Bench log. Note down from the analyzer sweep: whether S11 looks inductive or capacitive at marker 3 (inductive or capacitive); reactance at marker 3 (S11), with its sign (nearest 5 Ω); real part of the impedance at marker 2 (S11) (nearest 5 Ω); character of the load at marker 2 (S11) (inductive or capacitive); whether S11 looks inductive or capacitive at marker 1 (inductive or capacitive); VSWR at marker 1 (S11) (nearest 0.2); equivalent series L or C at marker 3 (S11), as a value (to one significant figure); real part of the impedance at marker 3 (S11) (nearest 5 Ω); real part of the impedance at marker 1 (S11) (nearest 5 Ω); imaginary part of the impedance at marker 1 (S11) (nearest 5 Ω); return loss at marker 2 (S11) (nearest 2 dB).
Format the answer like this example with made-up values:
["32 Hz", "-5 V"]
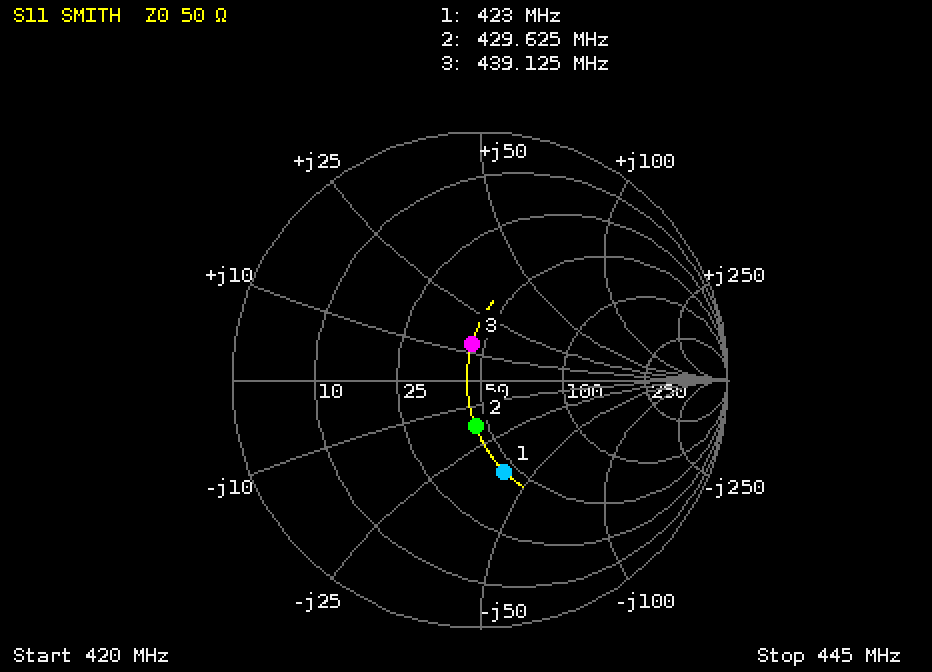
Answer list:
["inductive", "+15 Ω", "45 Ω", "capacitive", "capacitive", "2.2", "5 nH", "45 Ω", "45 Ω", "-40 Ω", "14 dB"]
